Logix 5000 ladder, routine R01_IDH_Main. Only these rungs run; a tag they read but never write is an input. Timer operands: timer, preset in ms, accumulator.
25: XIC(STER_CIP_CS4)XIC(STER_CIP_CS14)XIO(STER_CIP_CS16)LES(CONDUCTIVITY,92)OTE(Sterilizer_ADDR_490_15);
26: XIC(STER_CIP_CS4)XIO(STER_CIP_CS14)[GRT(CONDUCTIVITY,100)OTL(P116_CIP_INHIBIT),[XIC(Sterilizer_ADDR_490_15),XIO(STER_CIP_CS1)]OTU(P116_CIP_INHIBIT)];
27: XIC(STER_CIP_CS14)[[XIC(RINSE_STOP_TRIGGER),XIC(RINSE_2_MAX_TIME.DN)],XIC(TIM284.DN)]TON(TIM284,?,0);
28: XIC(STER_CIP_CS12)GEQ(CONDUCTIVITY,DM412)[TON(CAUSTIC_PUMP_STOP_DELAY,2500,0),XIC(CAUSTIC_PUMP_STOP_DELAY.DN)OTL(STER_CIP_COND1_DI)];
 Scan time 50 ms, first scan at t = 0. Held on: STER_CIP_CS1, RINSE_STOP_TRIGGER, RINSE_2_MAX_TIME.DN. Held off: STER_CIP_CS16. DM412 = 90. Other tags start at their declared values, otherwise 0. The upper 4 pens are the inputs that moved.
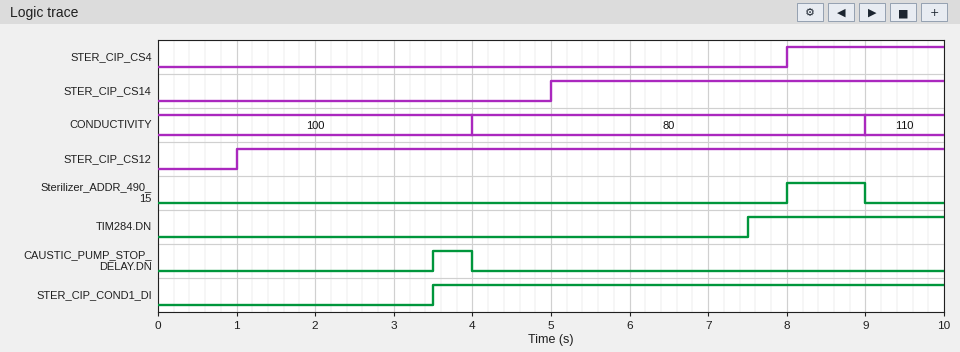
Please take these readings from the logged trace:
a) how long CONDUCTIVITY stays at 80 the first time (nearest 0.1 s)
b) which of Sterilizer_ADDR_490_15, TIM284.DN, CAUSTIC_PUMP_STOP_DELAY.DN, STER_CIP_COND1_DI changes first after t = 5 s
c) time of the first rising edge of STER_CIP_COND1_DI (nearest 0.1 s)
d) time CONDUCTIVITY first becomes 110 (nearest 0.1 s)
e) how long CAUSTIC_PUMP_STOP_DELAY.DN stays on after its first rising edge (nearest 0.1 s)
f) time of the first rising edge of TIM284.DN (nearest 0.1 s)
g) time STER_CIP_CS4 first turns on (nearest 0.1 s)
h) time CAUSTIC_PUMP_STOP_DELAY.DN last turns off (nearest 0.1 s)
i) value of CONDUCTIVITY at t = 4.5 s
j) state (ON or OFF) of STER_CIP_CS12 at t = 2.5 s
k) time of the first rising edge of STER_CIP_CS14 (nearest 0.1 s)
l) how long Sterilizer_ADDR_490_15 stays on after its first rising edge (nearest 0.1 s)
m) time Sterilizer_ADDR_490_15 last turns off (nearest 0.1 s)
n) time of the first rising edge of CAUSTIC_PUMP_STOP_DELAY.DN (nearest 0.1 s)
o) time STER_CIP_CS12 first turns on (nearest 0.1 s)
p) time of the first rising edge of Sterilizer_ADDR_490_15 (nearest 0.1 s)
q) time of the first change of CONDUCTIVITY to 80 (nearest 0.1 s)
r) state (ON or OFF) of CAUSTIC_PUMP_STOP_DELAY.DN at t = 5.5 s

5.0 s
TIM284.DN
3.5 s
9.0 s
0.5 s
7.5 s
8.0 s
4.0 s
80
ON
5.0 s
1.0 s
9.0 s
3.5 s
1.0 s
8.0 s
4.0 s
OFF
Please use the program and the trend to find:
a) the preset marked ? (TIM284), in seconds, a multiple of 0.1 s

2.5 s
